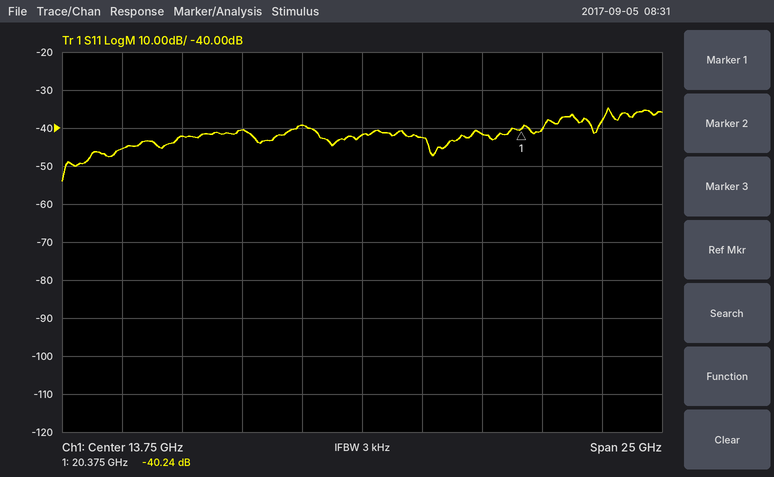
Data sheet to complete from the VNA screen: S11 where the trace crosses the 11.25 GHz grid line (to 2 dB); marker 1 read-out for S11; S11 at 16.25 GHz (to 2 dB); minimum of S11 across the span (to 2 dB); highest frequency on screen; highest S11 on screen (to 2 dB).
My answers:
-40 dB
-40.24 dB
-42 dB
-54 dB
26.25 GHz
-34 dB
